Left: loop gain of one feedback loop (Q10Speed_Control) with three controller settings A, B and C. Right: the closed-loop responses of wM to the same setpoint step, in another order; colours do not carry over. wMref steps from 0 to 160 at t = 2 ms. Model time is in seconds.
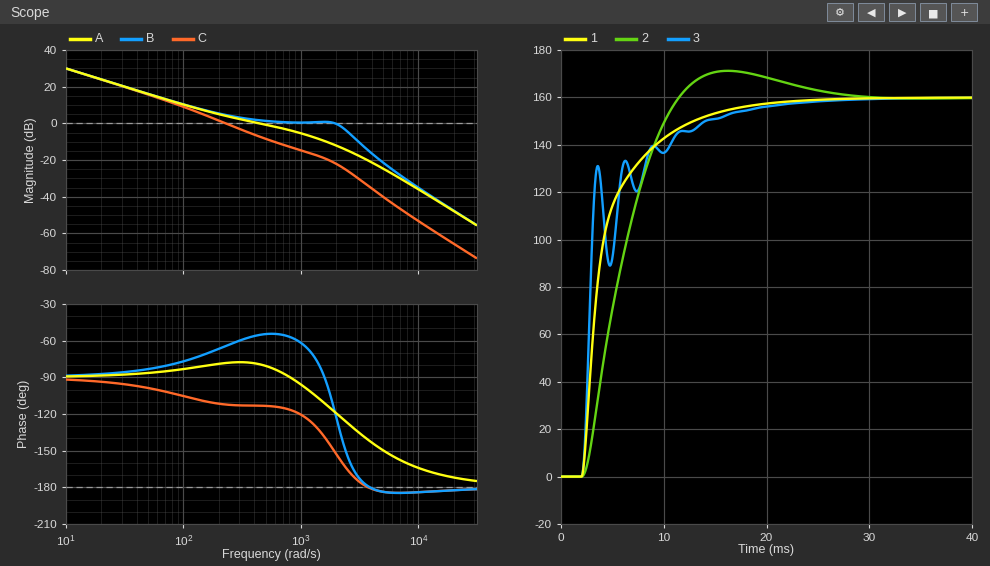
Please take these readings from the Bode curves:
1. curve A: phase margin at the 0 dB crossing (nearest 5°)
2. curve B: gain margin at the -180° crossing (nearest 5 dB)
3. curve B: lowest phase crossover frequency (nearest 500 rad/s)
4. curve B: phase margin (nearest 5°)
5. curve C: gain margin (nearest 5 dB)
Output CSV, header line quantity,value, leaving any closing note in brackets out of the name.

quantity,value
curve A: phase margin at the 0 dB crossing,100°
curve B: gain margin at the -180° crossing,15 dB
curve B: lowest phase crossover frequency,4000 rad/s
curve B: phase margin,60°
curve C: gain margin,35 dB
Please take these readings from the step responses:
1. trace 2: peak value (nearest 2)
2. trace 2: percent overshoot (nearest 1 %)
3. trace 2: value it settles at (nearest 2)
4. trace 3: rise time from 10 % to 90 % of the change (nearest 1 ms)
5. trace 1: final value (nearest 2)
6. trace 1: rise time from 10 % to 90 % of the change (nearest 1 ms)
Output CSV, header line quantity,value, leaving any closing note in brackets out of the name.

quantity,value
trace 2: peak value,172
trace 2: percent overshoot,7 %
trace 2: value it settles at,160
trace 3: rise time from 10 % to 90 % of the change,9 ms
trace 1: final value,160
trace 1: rise time from 10 % to 90 % of the change,8 ms
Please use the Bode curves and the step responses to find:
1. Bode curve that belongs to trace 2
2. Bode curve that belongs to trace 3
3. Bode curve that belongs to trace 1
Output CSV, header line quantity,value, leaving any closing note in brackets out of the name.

quantity,value
Bode curve that belongs to trace 2,C
Bode curve that belongs to trace 3,B
Bode curve that belongs to trace 1,A
